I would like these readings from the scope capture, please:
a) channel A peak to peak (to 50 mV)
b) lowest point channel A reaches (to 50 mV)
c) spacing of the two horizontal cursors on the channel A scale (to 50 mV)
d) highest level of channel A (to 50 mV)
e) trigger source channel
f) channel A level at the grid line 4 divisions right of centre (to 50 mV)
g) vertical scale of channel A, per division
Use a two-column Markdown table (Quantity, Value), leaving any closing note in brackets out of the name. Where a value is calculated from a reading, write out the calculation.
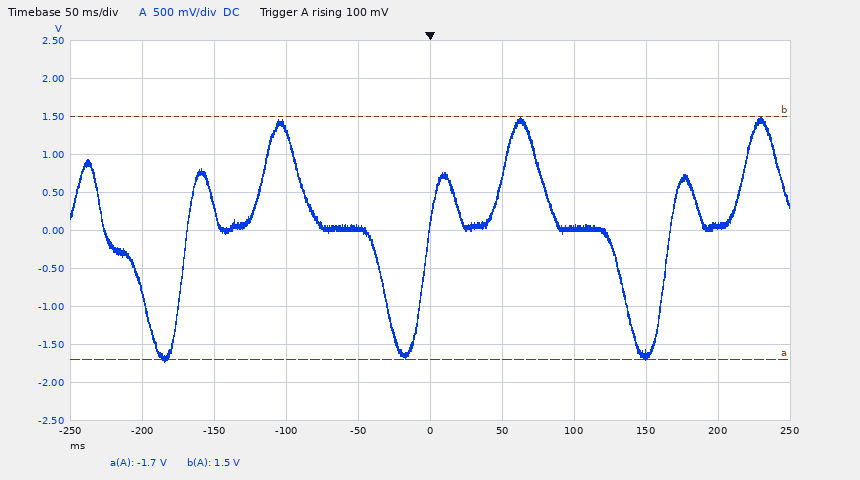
| Quantity | Value |
|---|---|
| channel A peak to peak | 1.50 V − (-1.70 V) = 3.20 V |
| lowest point channel A reaches | -1.70 V |
| spacing of the two horizontal cursors on the channel A scale | 3.20 V |
| highest level of channel A | 1.50 V |
| trigger source channel | channel A |
| channel A level at the grid line 4 divisions right of centre | 50 mV |
| vertical scale of channel A, per division | 500 mV |
